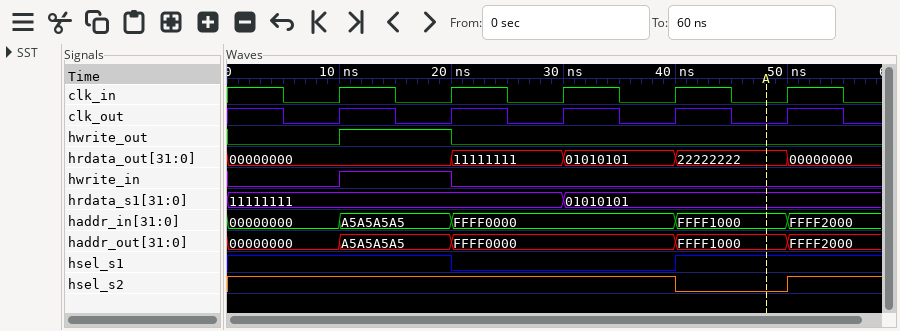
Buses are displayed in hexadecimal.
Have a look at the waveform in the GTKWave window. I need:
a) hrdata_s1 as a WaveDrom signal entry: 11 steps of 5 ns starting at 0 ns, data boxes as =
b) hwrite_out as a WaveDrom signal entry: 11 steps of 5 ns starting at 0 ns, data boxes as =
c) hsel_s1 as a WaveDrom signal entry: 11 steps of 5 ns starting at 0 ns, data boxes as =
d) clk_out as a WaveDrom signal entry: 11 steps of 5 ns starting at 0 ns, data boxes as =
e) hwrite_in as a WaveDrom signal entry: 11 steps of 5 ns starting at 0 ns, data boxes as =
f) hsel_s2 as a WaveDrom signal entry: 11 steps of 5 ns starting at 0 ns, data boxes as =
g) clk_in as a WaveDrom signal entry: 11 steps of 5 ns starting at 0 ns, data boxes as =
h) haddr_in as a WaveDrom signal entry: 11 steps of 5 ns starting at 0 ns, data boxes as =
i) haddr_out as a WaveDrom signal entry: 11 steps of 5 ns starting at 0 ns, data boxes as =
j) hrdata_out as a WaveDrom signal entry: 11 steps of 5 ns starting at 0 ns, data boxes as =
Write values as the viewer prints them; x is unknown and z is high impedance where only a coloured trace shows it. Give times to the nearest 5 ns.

{name: 'hrdata_s1', wave: '=.....=....', data: '11111111 01010101'}
{name: 'hwrite_out', wave: '0.1.0......'}
{name: 'hsel_s1', wave: '1...0...1..'}
{name: 'clk_out', wave: '10101010101'}
{name: 'hwrite_in', wave: '0.1.0......'}
{name: 'hsel_s2', wave: '1.......0.1'}
{name: 'clk_in', wave: '10101010101'}
{name: 'haddr_in', wave: '=.=.=...=.=', data: '00000000 A5A5A5A5 FFFF0000 FFFF1000 FFFF2000'}
{name: 'haddr_out', wave: '=.=.=...=.=', data: '00000000 A5A5A5A5 FFFF0000 FFFF1000 FFFF2000'}
{name: 'hrdata_out', wave: '=...=.=.=.=', data: '00000000 11111111 01010101 22222222 00000000'}
